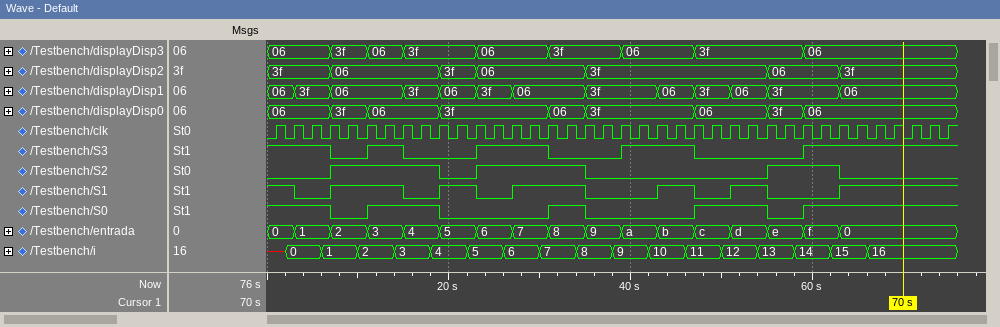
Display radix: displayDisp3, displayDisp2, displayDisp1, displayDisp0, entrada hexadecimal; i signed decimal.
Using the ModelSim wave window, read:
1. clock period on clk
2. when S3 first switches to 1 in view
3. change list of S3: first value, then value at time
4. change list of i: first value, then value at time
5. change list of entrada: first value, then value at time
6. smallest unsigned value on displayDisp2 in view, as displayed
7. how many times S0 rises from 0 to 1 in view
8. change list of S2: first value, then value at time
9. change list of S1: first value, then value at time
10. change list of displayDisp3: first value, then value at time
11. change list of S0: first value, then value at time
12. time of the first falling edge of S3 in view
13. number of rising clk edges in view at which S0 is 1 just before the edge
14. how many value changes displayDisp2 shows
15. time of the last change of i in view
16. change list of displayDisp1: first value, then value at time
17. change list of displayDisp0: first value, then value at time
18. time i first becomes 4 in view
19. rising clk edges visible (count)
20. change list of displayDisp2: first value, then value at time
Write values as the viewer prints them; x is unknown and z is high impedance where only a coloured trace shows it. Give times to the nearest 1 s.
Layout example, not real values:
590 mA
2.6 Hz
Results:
2 s
11 s
1, 0 at 7 s, 1 at 11 s, 0 at 15 s, 1 at 23 s, 0 at 31 s, 1 at 39 s, 0 at 47 s, 1 at 59 s
x, 0 at 2 s, 1 at 6 s, 2 at 10 s, 3 at 14 s, 4 at 18 s, 5 at 22 s, 6 at 26 s, 7 at 30 s, 8 at 34 s, 9 at 38 s, 10 at 42 s, 11 at 46 s, 12 at 50 s, 13 at 54 s, 14 at 58 s, 15 at 62 s, 16 at 66 s
0, 1 at 3 s, 2 at 7 s, 3 at 11 s, 4 at 15 s, 5 at 19 s, 6 at 23 s, 7 at 27 s, 8 at 31 s, 9 at 35 s, a at 39 s, b at 43 s, c at 47 s, d at 51 s, e at 55 s, f at 59 s, 0 at 63 s
06
4
0, 1 at 7 s, 0 at 19 s, 1 at 23 s, 0 at 35 s, 1 at 55 s, 0 at 63 s
1, 0 at 3 s, 1 at 7 s, 0 at 15 s, 1 at 19 s, 0 at 23 s, 1 at 27 s, 0 at 35 s, 1 at 43 s, 0 at 47 s, 1 at 51 s, 0 at 55 s, 1 at 63 s
06, 3f at 7 s, 06 at 11 s, 3f at 15 s, 06 at 23 s, 3f at 31 s, 06 at 39 s, 3f at 47 s, 06 at 59 s
1, 0 at 7 s, 1 at 11 s, 0 at 19 s, 1 at 31 s, 0 at 35 s, 1 at 47 s, 0 at 55 s, 1 at 59 s
7 s
22
6
66 s
06, 3f at 3 s, 06 at 7 s, 3f at 15 s, 06 at 19 s, 3f at 23 s, 06 at 27 s, 3f at 35 s, 06 at 43 s, 3f at 47 s, 06 at 51 s, 3f at 55 s, 06 at 63 s
06, 3f at 7 s, 06 at 11 s, 3f at 19 s, 06 at 31 s, 3f at 35 s, 06 at 47 s, 3f at 55 s, 06 at 59 s
18 s
38
3f, 06 at 7 s, 3f at 19 s, 06 at 23 s, 3f at 35 s, 06 at 55 s, 3f at 63 s
